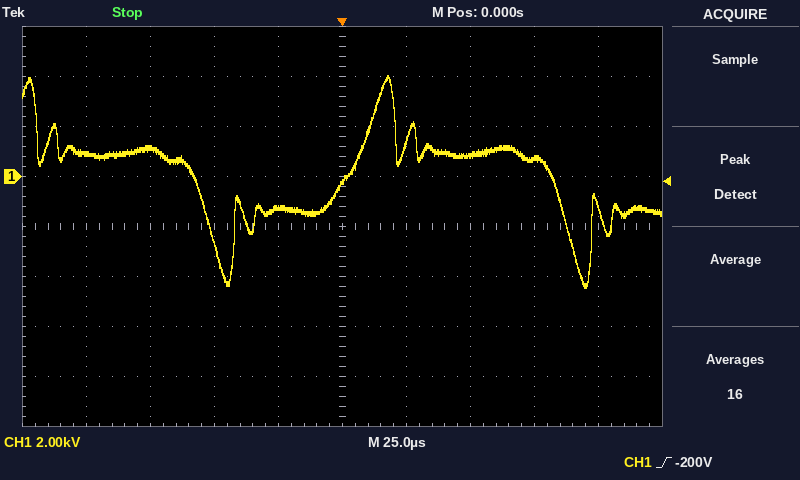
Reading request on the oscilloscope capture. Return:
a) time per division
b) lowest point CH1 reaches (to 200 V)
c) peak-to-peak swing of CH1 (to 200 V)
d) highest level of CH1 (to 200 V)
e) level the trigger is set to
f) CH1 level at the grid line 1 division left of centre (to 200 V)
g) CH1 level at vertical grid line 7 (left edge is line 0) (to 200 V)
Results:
25 µs
-4.4 kV
8.4 kV
4.0 kV
-200 V
-1.2 kV
800 V
